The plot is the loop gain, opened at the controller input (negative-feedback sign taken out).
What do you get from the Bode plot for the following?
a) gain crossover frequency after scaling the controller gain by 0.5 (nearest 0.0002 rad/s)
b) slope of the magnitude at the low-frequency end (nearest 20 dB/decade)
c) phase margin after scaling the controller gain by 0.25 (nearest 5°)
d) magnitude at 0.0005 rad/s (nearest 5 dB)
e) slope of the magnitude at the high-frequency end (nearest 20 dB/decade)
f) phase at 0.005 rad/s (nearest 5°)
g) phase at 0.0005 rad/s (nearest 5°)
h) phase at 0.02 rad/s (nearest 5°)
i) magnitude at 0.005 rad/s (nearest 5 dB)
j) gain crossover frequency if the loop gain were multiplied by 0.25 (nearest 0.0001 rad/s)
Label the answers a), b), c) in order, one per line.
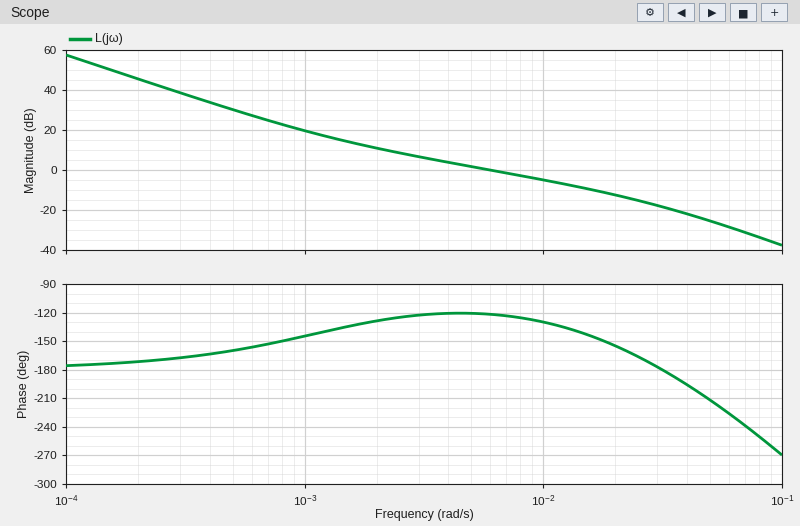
a) 0.0032 rad/s
b) -40 dB/decade
c) 50°
d) 30 dB
e) -40 dB/decade
f) -120°
g) -160°
h) -155°
i) 0 dB
j) 0.0018 rad/s
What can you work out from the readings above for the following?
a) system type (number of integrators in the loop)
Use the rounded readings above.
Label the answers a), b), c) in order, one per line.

a) 2
